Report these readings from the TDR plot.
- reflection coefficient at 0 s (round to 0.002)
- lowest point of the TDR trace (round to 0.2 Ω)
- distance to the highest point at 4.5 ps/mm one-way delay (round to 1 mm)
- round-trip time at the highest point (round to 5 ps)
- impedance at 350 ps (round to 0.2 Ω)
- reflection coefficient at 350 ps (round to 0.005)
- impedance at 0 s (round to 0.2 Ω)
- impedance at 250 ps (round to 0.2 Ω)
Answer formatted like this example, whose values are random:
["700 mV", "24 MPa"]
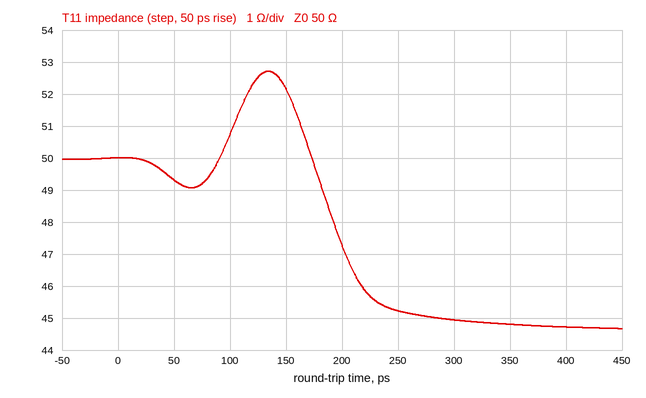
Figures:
["0.000", "44.6 Ω", "15 mm", "135 ps", "44.8 Ω", "-0.055", "50.0 Ω", "45.2 Ω"]
